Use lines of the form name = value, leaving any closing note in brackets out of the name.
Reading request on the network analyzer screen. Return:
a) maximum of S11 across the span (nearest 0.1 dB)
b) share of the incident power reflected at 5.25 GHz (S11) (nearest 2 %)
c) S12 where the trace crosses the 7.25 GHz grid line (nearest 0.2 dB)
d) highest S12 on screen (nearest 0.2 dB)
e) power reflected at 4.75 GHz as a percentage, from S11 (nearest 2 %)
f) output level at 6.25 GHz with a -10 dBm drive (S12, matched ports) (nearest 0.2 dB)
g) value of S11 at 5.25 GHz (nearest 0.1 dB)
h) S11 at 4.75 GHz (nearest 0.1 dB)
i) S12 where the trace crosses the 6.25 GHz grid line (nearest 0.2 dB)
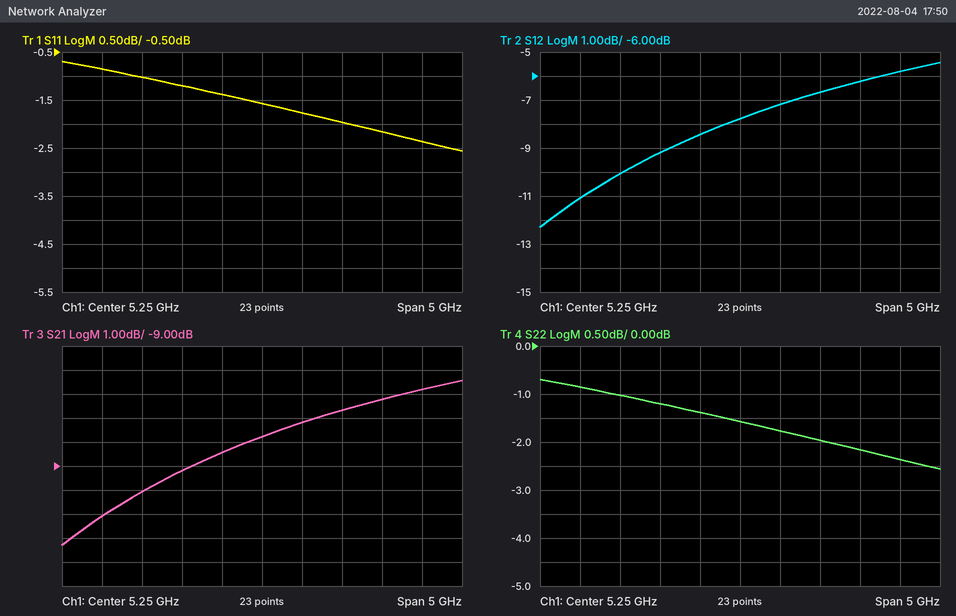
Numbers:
maximum of S11 across the span = -0.7 dB
share of the incident power reflected at 5.25 GHz (S11) = 70 %
S12 where the trace crosses the 7.25 GHz grid line = -5.8 dB
highest S12 on screen = -5.4 dB
power reflected at 4.75 GHz as a percentage, from S11 = 72 %
output level at 6.25 GHz with a -10 dBm drive (S12, matched ports) = -16.6 dBm
value of S11 at 5.25 GHz = -1.6 dB
S11 at 4.75 GHz = -1.4 dB
S12 where the trace crosses the 6.25 GHz grid line = -6.6 dB
